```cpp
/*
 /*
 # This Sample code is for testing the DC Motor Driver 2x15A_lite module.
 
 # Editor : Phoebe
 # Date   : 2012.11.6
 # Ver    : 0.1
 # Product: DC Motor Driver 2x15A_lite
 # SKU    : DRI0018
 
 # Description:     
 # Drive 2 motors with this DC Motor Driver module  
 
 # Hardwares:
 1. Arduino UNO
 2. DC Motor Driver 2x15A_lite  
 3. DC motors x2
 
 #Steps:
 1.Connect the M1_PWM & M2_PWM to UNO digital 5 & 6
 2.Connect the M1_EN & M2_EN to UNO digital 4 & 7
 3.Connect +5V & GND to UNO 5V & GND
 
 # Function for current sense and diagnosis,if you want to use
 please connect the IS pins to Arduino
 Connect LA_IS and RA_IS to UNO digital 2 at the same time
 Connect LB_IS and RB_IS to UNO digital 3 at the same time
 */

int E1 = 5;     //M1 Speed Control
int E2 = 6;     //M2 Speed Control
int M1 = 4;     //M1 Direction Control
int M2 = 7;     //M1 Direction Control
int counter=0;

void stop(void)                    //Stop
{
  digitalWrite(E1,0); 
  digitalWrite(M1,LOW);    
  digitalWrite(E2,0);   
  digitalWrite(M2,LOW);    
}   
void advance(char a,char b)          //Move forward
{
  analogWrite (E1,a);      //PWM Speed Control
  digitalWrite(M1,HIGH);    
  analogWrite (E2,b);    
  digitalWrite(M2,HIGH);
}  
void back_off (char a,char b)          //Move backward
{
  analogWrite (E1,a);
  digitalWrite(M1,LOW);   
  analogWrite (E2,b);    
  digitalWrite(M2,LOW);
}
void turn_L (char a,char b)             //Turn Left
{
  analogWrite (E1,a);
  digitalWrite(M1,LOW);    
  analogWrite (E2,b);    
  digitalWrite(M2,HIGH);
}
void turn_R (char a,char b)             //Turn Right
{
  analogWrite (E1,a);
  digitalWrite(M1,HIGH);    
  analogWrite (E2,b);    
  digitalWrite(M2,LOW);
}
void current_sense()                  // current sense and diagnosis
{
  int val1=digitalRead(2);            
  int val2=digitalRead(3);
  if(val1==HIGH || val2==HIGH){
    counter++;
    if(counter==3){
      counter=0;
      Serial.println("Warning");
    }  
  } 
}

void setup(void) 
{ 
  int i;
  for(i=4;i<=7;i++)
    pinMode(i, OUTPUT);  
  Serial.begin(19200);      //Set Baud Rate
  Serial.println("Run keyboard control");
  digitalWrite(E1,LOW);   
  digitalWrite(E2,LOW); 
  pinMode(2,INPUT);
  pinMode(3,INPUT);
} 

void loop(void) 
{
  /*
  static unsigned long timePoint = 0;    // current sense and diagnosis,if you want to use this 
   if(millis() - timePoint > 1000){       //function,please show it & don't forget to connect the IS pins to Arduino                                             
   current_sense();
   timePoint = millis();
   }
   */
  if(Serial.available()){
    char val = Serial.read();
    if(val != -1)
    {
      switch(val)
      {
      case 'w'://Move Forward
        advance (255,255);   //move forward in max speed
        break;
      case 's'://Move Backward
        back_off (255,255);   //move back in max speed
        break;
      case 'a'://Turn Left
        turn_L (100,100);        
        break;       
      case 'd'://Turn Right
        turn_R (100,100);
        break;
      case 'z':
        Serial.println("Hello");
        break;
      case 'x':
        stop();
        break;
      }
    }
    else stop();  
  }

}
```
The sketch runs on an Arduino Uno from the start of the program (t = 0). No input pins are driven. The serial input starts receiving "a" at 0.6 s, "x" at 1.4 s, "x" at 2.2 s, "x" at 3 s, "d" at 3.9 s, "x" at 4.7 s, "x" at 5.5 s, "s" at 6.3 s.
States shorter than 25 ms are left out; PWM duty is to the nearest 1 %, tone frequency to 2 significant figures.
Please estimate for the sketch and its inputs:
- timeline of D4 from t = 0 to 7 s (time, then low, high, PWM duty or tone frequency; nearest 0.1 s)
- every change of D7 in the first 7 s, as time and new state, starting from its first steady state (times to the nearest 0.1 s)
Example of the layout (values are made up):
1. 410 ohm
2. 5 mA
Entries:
1. 0 s low; 3.9 s high; 4.7 s low
2. 0 s low; 0.6 s high; 1.4 s low
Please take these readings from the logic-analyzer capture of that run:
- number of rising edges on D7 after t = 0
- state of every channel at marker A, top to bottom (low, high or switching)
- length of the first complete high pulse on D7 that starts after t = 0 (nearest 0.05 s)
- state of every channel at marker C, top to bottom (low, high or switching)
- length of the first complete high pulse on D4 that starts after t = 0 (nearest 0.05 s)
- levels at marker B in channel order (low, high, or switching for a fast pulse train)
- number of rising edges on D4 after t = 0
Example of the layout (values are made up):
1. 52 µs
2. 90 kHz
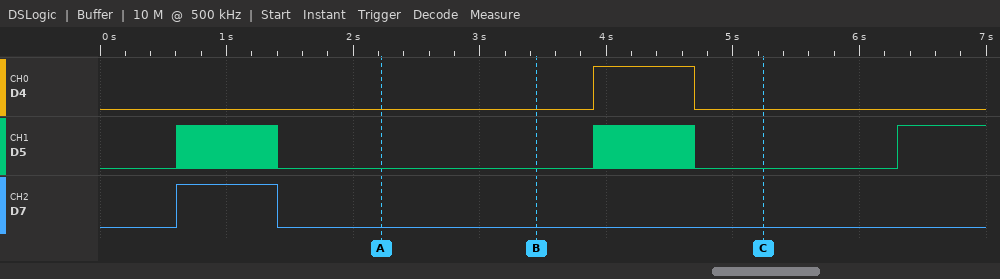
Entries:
1. 1
2. D4 low, D5 low, D7 low
3. 0.80 s
4. D4 low, D5 low, D7 low
5. 0.80 s
6. D4 low, D5 low, D7 low
7. 1
